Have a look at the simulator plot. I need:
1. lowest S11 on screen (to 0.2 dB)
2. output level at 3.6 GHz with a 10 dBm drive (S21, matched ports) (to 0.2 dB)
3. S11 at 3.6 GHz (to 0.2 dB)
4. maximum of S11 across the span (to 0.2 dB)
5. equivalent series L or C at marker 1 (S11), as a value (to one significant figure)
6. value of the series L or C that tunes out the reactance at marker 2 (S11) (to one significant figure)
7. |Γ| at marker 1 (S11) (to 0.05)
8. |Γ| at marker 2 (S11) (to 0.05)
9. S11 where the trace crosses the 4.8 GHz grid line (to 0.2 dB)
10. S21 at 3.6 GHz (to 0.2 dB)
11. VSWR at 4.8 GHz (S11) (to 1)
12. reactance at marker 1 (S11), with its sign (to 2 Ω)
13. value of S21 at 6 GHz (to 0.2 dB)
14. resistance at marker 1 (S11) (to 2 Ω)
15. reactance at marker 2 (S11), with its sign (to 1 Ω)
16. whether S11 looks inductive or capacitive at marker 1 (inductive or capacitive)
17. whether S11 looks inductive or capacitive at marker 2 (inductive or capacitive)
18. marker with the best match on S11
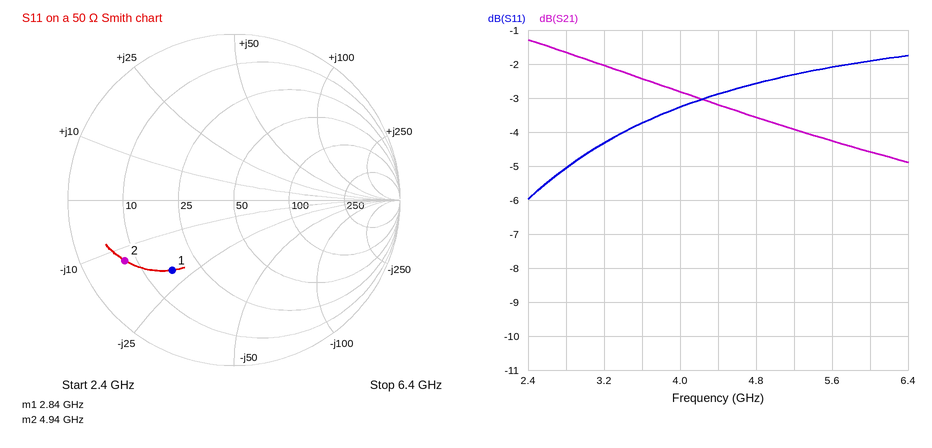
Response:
-6.0 dB
7.6 dBm
-3.8 dB
-1.8 dB
3 pF
400 pH
0.55
0.75
-2.6 dB
-2.4 dB
7
-20 Ω
-4.6 dB
16 Ω
-13 Ω
capacitive
capacitive
marker 1
